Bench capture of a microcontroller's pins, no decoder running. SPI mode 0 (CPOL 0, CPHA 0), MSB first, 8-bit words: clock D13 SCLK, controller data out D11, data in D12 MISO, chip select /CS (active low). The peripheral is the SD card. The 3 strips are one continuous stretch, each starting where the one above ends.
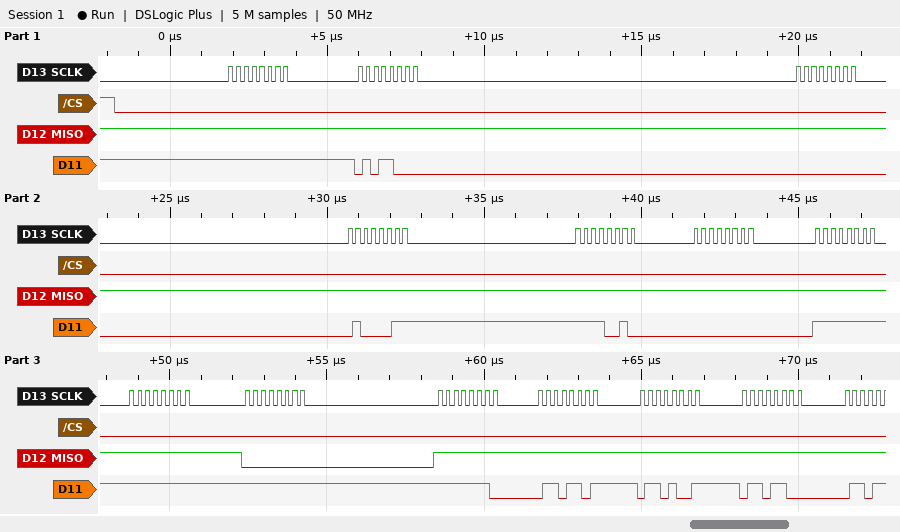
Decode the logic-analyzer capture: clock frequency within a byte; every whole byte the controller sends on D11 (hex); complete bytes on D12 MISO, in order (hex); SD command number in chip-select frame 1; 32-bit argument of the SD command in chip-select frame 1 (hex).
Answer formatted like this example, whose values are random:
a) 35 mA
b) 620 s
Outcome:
a) 4 MHz
b) FF 58 00 43 F2 00 FF FF FF FE 6D 69 6C
c) FF FF FF FF FF FF FF FF 00 FF FF FF FF
d) CMD24
e) 0x0043F200
